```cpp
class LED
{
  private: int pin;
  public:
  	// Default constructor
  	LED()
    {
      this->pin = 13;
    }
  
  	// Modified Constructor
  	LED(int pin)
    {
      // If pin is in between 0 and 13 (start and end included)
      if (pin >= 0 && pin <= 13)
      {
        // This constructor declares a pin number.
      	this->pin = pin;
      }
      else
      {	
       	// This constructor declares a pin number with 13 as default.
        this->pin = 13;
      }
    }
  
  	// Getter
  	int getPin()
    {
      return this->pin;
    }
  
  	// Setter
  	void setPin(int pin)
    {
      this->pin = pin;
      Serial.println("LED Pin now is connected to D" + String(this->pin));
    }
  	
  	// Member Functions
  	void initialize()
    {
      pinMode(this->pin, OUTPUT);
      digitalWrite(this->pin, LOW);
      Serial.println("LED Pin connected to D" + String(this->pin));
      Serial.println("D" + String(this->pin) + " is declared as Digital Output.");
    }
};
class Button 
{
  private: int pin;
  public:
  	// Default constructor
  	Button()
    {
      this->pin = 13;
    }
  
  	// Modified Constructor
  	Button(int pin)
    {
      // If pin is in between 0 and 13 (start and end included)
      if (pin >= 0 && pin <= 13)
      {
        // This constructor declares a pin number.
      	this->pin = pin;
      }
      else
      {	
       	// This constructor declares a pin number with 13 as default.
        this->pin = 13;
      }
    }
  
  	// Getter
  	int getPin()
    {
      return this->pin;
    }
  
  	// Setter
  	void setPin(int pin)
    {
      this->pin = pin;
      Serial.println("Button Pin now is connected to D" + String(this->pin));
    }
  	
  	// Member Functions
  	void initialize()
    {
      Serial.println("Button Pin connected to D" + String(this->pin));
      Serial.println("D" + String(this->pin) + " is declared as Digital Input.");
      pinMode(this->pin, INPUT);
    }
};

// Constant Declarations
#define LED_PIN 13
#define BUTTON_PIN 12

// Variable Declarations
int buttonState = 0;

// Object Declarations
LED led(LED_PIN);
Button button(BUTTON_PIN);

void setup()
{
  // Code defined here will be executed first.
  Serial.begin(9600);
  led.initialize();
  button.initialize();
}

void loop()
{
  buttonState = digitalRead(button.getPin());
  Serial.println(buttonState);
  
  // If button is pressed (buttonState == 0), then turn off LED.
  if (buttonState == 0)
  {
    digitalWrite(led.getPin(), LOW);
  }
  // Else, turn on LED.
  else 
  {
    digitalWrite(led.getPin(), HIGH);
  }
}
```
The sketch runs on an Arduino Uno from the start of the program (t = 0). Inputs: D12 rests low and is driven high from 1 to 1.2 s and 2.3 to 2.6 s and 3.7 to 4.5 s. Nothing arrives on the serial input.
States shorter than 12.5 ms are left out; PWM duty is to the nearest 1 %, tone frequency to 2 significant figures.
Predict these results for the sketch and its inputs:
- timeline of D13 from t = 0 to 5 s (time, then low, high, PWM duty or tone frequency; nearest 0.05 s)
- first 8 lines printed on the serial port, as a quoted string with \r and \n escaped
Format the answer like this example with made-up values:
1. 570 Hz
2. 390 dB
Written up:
1. 0 s low; 1 s high; 1.2 s low; 2.3 s high; 2.6 s low; 3.7 s high; 4.5 s low
2. "LED Pin connected to D13\r\nD13 is declared as Digital Output.\r\nButton Pin connected to D12\r\nD12 is declared as Digital Input.\r\n0\r\n0\r\n0\r\n0\r\n"
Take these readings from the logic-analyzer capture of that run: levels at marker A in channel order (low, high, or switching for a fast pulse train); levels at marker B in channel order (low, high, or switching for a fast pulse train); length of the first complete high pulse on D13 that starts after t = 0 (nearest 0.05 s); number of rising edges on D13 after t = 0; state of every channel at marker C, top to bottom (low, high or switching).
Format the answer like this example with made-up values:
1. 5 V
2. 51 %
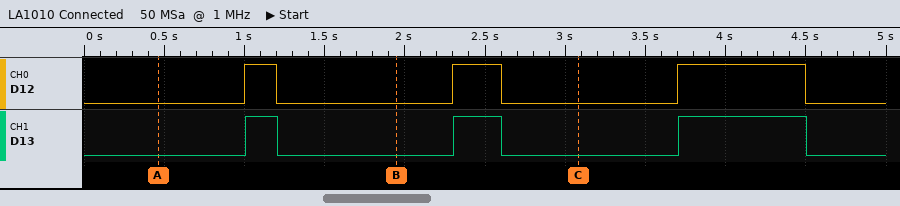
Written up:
1. D12 low, D13 low
2. D12 low, D13 low
3. 0.20 s
4. 3
5. D12 low, D13 low
